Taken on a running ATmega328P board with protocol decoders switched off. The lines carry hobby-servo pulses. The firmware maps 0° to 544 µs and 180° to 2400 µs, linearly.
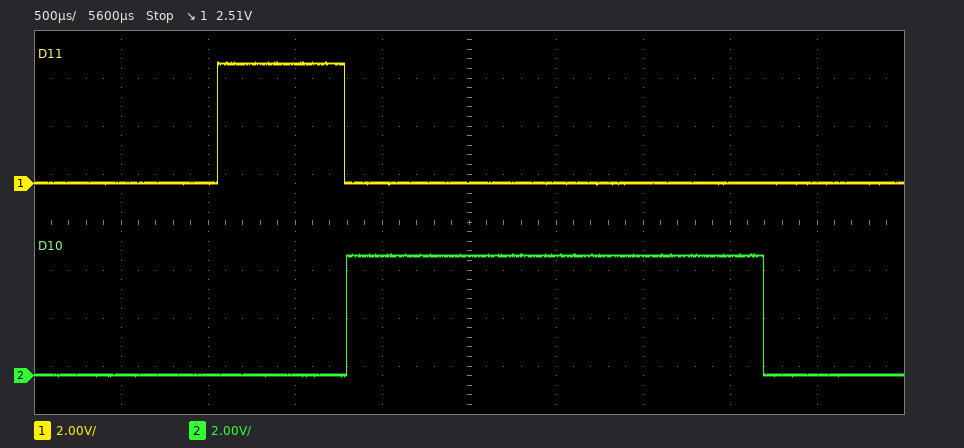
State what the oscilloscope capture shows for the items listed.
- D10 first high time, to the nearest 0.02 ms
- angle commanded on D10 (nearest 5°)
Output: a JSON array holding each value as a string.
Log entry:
["2.40 ms", "180°"]
